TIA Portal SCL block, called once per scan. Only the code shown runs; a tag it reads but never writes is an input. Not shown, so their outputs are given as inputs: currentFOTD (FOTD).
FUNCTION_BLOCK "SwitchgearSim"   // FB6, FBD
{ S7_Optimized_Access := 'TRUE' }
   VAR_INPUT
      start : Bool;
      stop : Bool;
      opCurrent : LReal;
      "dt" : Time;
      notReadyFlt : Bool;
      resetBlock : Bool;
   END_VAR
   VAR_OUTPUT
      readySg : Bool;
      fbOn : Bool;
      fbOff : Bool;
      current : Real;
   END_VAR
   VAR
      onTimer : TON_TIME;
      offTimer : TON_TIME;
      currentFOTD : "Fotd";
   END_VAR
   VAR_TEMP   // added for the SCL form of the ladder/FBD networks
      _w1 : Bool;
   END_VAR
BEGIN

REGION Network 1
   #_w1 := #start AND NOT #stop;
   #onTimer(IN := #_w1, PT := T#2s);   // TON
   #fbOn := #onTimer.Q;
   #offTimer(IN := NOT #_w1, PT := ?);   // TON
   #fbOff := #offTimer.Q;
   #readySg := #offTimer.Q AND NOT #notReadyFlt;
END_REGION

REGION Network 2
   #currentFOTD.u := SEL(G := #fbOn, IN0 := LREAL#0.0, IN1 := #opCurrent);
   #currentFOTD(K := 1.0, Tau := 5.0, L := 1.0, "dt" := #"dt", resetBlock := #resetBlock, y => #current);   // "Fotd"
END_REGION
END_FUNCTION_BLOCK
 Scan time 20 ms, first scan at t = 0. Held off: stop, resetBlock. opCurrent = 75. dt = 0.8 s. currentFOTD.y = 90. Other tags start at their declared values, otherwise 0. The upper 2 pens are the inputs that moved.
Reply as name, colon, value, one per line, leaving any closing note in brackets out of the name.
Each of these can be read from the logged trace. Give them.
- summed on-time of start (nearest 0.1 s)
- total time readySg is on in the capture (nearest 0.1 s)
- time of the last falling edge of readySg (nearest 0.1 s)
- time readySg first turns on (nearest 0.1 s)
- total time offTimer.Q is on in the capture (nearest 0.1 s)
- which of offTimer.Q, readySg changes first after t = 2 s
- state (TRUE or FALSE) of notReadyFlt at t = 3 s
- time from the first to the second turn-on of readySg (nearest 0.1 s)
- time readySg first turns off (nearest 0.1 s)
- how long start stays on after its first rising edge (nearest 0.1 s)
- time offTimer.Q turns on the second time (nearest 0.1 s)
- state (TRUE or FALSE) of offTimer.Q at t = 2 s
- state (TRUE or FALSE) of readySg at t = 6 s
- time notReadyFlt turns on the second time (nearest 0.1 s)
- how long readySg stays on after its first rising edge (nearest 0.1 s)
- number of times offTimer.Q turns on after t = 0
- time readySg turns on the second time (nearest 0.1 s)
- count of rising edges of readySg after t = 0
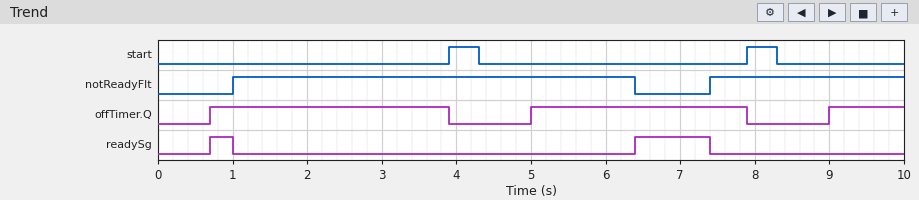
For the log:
summed on-time of start: 0.8 s
total time readySg is on in the capture: 1.3 s
time of the last falling edge of readySg: 7.4 s
time readySg first turns on: 0.7 s
total time offTimer.Q is on in the capture: 7.1 s
which of offTimer.Q, readySg changes first after t = 2 s: offTimer.Q
state (TRUE or FALSE) of notReadyFlt at t = 3 s: TRUE
time from the first to the second turn-on of readySg: 5.7 s
time readySg first turns off: 1.0 s
how long start stays on after its first rising edge: 0.4 s
time offTimer.Q turns on the second time: 5.0 s
state (TRUE or FALSE) of offTimer.Q at t = 2 s: TRUE
state (TRUE or FALSE) of readySg at t = 6 s: FALSE
time notReadyFlt turns on the second time: 7.4 s
how long readySg stays on after its first rising edge: 0.3 s
number of times offTimer.Q turns on after t = 0: 3
time readySg turns on the second time: 6.4 s
count of rising edges of readySg after t = 0: 2
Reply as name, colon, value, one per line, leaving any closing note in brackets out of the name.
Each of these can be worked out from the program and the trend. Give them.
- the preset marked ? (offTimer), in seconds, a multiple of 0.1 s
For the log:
the preset marked ? (offTimer), in seconds, a multiple of 0.1 s: 0.7 s
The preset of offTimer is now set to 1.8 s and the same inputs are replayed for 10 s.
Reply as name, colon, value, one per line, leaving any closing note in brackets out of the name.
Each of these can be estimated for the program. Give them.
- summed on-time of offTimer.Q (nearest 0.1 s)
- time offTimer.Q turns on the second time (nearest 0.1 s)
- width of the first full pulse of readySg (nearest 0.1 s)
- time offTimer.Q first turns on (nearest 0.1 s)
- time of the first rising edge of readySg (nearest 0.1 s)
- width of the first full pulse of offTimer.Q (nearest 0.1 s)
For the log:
summed on-time of offTimer.Q: 3.9 s
time offTimer.Q turns on the second time: 6.1 s
width of the first full pulse of readySg: 1.0 s
time offTimer.Q first turns on: 1.8 s
time of the first rising edge of readySg: 6.4 s
width of the first full pulse of offTimer.Q: 2.1 s
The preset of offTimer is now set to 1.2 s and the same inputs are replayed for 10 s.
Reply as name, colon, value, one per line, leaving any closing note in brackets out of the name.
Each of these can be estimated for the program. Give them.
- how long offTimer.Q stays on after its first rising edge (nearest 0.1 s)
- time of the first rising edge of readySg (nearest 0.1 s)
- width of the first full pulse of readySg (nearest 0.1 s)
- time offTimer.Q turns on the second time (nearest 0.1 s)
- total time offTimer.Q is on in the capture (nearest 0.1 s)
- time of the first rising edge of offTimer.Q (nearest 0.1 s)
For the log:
how long offTimer.Q stays on after its first rising edge: 2.7 s
time of the first rising edge of readySg: 6.4 s
width of the first full pulse of readySg: 1.0 s
time offTimer.Q turns on the second time: 5.5 s
total time offTimer.Q is on in the capture: 5.6 s
time of the first rising edge of offTimer.Q: 1.2 s
